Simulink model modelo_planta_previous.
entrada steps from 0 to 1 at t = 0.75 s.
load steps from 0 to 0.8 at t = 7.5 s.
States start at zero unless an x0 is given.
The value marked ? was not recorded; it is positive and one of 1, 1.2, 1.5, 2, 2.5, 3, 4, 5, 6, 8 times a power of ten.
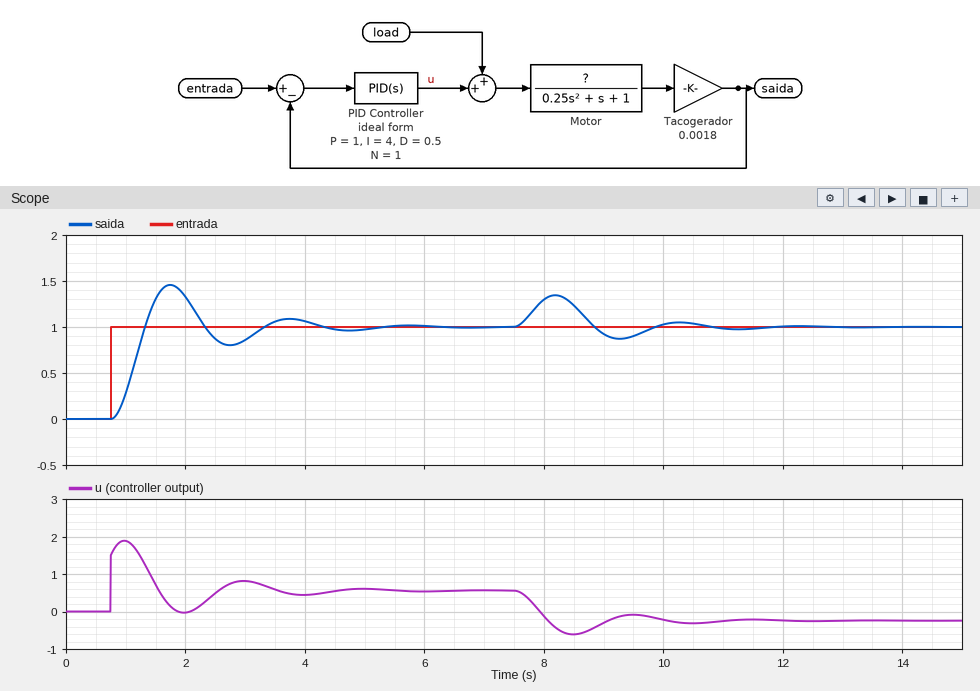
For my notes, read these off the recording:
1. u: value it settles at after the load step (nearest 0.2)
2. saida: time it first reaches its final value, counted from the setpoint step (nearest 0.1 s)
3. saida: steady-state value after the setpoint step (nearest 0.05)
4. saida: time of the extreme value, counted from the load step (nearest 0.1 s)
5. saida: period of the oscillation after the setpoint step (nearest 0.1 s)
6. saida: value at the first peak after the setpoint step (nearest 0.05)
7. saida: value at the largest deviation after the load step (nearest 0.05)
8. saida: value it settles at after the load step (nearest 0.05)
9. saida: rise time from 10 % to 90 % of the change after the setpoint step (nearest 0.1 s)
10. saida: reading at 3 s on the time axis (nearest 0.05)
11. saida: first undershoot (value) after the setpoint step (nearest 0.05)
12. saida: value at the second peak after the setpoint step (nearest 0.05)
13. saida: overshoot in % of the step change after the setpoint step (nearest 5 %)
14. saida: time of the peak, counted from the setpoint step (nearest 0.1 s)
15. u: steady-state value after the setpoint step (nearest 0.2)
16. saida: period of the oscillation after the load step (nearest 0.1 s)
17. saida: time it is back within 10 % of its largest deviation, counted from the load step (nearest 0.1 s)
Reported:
-0.2
0.6 s
1.00
0.7 s
2.0 s
1.45
1.35
1.00
0.4 s
0.85
0.80
1.10
45 %
1.0 s
0.6
2.1 s
3.0 s
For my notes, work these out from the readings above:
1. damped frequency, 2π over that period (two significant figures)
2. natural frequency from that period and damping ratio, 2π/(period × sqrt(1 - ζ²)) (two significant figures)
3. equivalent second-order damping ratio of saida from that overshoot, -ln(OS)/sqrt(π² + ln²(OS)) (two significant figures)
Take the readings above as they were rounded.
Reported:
3.1 rad/s
3.2 rad/s
0.25
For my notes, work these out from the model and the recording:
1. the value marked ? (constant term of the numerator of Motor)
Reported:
1000
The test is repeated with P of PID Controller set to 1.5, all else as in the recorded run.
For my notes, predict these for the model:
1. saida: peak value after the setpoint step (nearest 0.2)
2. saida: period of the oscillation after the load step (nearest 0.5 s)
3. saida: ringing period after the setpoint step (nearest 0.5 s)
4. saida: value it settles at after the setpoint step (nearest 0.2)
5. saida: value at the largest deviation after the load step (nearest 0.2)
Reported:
1.6
1.5 s
1.5 s
1.0
1.2
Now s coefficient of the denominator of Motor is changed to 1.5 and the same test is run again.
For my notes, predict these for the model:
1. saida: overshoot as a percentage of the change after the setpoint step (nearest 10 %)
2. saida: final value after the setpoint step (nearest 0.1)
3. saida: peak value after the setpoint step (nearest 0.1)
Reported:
40 %
1.0
1.4
